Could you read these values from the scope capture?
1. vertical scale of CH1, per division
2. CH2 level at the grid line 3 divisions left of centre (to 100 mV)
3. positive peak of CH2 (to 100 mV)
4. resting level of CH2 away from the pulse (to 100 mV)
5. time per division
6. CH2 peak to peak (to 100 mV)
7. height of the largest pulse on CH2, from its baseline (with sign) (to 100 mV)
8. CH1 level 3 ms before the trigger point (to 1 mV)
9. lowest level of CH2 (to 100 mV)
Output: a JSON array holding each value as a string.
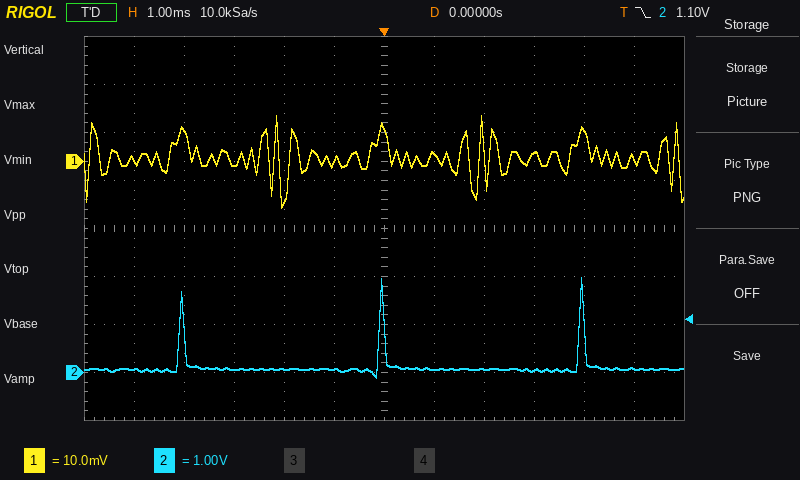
["10 mV", "100 mV", "2.0 V", "100 mV", "1 ms", "2.1 V", "+1.9 V", "-1 mV", "-100 mV"]
